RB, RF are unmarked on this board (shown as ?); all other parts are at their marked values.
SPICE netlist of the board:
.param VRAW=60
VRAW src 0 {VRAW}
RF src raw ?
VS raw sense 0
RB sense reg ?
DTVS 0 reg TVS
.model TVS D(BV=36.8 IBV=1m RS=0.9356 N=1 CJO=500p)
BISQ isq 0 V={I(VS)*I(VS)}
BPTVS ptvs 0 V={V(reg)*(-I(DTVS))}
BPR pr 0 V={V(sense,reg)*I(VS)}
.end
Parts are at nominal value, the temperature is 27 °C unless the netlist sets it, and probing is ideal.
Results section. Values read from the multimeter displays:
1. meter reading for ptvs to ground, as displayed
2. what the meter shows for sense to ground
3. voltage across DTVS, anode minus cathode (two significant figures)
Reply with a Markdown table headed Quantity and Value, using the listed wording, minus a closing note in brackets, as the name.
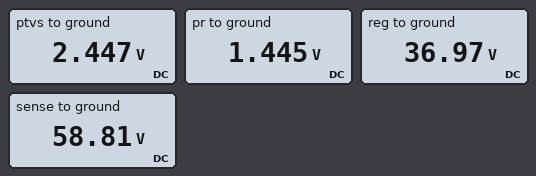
| Quantity | Value |
|---|---|
| meter reading for ptvs to ground, as displayed | 2.447 V |
| what the meter shows for sense to ground | 58.81 V |
| voltage across DTVS, anode minus cathode | -37 V |
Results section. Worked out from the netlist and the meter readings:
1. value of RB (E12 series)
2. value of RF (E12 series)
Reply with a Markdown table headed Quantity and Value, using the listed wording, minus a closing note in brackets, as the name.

| Quantity | Value |
|---|---|
| value of RB | 330 Ω |
| value of RF | 18 Ω |
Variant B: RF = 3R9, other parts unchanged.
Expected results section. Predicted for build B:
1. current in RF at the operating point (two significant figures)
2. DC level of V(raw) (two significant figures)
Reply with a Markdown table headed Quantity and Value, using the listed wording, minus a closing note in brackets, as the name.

| Quantity | Value |
|---|---|
| current in RF at the operating point | 69 mA |
| DC level of V(raw) | 60 V |
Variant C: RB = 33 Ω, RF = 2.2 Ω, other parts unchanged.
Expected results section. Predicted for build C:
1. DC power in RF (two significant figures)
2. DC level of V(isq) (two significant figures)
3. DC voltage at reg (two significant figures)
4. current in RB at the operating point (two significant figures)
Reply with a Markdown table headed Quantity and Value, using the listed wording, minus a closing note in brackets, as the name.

| Quantity | Value |
|---|---|
| DC power in RF | 890 mW |
| DC level of V(isq) | 410 mV |
| DC voltage at reg | 38 V |
| current in RB at the operating point | 640 mA |
